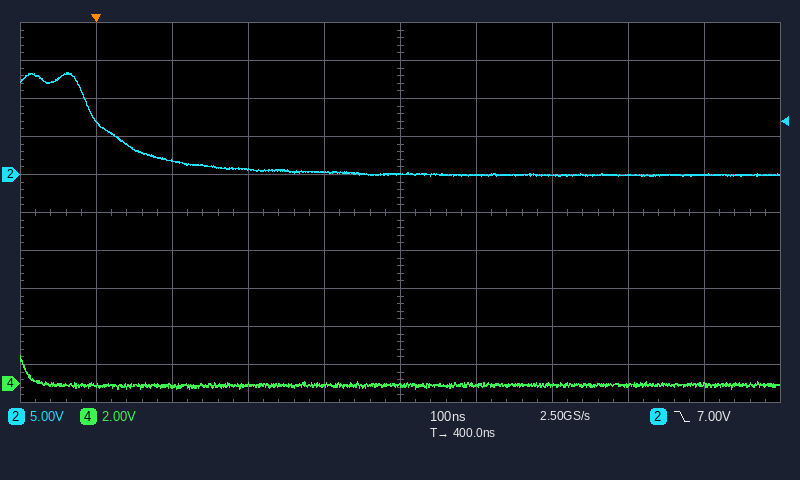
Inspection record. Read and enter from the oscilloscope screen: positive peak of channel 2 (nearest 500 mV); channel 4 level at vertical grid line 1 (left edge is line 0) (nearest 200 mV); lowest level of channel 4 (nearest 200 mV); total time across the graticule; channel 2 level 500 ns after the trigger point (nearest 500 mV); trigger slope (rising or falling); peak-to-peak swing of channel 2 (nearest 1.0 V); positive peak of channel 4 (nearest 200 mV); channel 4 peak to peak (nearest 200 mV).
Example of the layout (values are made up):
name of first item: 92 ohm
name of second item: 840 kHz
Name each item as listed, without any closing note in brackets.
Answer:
positive peak of channel 2: 13.5 V
channel 4 level at vertical grid line 1 (left edge is line 0): -200 mV
lowest level of channel 4: -400 mV
total time across the graticule: 1 µs
channel 2 level 500 ns after the trigger point: 0.0 V
trigger slope: falling
peak-to-peak swing of channel 2: 14.0 V
positive peak of channel 4: 1.4 V
channel 4 peak to peak: 1.8 V
